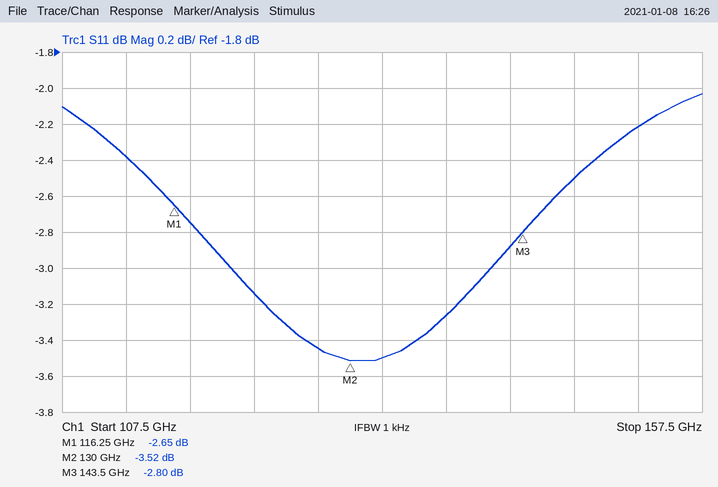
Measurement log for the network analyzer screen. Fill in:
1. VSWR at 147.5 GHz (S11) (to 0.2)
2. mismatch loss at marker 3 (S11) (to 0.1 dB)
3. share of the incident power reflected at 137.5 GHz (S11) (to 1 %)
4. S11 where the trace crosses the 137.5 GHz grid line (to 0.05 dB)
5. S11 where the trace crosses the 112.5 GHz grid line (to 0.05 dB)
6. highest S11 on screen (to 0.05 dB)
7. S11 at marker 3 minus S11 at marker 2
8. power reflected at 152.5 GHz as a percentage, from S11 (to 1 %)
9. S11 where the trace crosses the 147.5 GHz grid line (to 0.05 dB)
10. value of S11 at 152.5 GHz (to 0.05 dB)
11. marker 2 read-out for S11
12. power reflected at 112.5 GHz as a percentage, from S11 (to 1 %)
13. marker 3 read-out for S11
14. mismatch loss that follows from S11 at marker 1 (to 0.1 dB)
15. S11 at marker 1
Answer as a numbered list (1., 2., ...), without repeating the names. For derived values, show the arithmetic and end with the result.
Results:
1. |Γ| = 10^(-2.5/20) = 0.7499; VSWR = (1 + 0.7499)/(1 − 0.7499) ≈ 7.0
2. −10 log10(1 − 10^(-2.8/10)) ≈ 3.2 dB
3. 10^(-3.25/10) ≈ 47 %
4. -3.25 dB
5. -2.40 dB
6. -2.05 dB
7. -2.8 − (-3.52) = 0.72 dB
8. 10^(-2.2/10) ≈ 60 %
9. -2.50 dB
10. -2.20 dB
11. -3.52 dB
12. 10^(-2.4/10) ≈ 58 %
13. -2.80 dB
14. −10 log10(1 − 10^(-2.65/10)) ≈ 3.4 dB
15. -2.65 dB
